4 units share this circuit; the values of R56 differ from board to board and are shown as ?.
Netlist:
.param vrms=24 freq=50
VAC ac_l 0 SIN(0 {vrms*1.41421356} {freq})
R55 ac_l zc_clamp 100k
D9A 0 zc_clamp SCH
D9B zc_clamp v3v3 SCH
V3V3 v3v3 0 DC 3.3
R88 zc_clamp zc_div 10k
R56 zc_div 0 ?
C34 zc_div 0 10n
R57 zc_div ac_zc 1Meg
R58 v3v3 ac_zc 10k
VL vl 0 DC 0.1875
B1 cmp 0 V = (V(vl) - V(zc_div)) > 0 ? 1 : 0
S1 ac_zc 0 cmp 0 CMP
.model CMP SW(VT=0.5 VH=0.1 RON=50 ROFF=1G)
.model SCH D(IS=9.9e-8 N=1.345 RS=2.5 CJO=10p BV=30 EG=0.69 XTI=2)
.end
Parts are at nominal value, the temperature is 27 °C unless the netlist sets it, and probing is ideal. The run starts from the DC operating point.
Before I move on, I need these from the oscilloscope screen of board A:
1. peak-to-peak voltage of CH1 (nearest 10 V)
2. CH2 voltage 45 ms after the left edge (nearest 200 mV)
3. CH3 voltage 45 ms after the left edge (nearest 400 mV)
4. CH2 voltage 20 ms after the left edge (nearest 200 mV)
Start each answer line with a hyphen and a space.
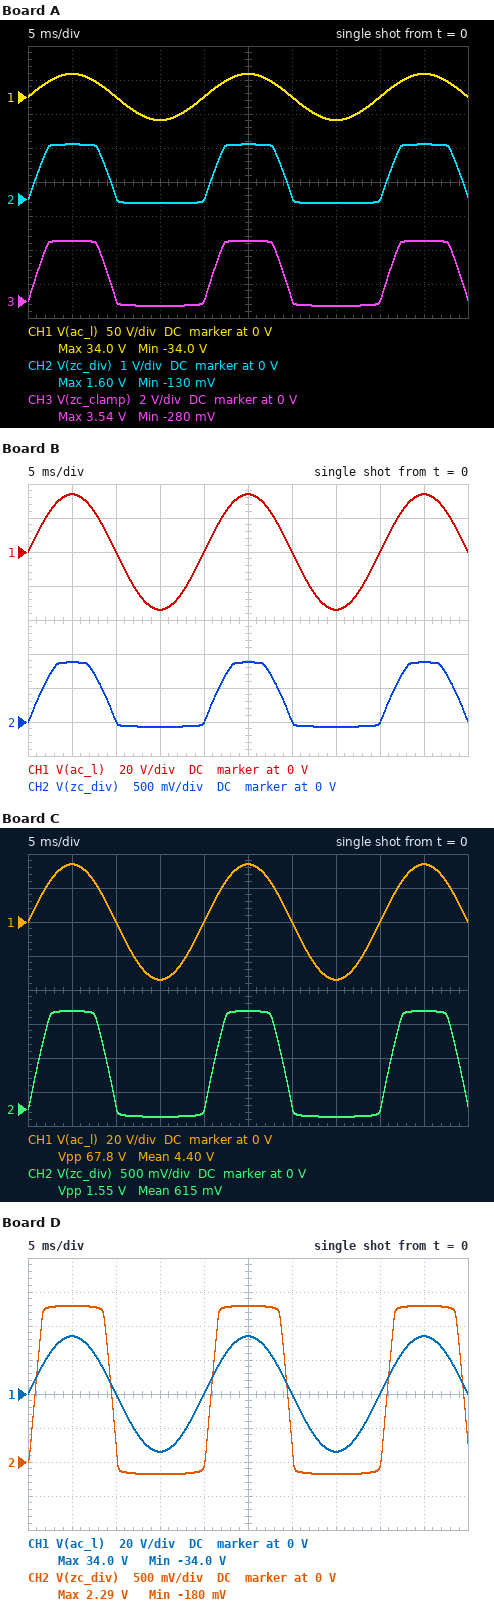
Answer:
- 70 V
- 1.6 V
- 3.6 V
- 0 V
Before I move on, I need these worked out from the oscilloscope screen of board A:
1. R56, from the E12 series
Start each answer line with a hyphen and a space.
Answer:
- 8.2 kΩ
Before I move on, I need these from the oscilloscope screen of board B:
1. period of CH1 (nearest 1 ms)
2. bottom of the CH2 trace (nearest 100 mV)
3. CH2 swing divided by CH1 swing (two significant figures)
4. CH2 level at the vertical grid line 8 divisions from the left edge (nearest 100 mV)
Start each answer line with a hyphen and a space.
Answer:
- 20 ms
- -100 mV
- 0.014
- 0 V
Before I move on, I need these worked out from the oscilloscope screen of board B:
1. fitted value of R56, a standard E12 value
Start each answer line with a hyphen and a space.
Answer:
- 3.3 kΩ
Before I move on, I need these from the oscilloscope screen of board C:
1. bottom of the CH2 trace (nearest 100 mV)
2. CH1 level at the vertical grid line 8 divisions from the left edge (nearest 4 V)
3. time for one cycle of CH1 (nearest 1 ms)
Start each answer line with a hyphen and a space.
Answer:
- -100 mV
- 0 V
- 20 ms
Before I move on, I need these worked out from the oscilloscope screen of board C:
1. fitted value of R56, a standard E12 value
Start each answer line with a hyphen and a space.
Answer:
- 6.8 kΩ
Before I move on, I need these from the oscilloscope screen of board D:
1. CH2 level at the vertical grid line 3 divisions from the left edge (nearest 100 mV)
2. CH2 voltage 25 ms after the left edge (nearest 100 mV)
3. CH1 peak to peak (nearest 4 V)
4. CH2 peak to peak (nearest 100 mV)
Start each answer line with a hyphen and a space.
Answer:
- -200 mV
- 2.3 V
- 68 V
- 2.5 V
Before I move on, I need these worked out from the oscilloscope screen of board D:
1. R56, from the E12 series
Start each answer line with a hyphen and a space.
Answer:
- 18 kΩ
